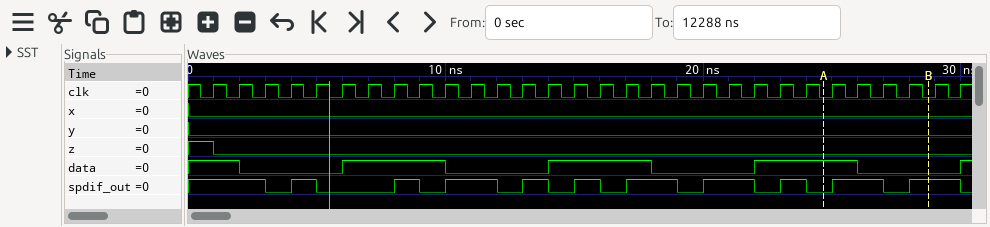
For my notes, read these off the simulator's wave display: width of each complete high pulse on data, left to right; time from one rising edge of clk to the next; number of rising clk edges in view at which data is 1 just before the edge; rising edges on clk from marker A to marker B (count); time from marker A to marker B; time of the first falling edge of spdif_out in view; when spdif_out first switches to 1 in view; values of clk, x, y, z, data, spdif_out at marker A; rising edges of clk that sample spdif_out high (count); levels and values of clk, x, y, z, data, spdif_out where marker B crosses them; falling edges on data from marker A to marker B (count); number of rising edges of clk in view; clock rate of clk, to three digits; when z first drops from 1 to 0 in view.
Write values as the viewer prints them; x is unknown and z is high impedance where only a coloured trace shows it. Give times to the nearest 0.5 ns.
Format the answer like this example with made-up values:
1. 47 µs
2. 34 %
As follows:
1. 4 ns, 4 ns, 4 ns
2. 1 ns
3. 14
4. 4
5. 4 ns
6. 3 ns
7. 4 ns
8. clk=0, x=0, y=0, z=0, data=1, spdif_out=0
9. 18
10. clk=0, x=0, y=0, z=0, data=0, spdif_out=1
11. 1
12. 30
13. 1.00 GHz
14. 1 ns
